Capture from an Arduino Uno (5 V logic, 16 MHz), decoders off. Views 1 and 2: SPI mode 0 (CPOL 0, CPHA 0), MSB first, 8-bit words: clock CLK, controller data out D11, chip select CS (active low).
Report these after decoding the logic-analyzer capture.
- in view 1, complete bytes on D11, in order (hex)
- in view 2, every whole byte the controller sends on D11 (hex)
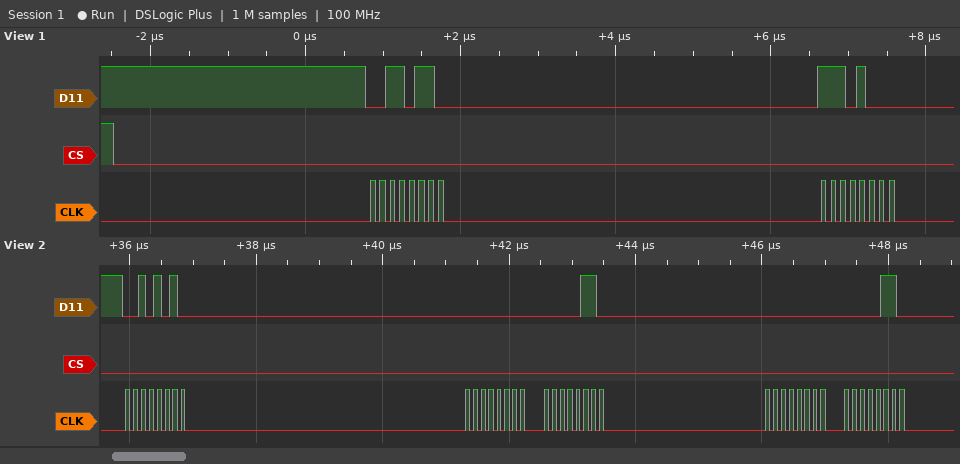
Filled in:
0x36 0xE8
2A 00 06 00 06
